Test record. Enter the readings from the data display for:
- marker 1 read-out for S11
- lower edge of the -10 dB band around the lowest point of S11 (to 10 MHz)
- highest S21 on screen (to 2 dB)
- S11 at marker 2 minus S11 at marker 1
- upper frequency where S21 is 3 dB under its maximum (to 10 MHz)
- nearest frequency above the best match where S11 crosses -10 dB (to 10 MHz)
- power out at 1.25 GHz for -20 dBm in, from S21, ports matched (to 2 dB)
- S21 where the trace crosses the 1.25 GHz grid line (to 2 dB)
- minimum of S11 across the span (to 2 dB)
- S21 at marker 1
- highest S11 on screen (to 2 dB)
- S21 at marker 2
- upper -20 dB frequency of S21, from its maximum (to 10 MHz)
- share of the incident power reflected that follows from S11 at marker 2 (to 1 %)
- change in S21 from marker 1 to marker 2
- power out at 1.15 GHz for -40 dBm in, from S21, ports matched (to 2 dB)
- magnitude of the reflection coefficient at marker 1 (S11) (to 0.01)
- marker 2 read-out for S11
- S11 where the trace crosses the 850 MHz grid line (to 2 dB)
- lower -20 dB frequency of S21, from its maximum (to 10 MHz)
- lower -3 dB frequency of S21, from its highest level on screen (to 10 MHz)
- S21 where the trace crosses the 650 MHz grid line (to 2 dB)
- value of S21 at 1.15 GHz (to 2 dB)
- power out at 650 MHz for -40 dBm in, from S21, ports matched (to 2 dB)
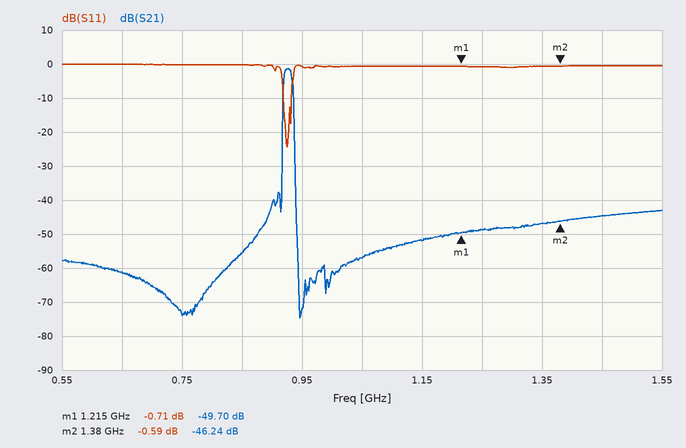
-0.71 dB
920 MHz
-2 dB
0.12 dB
930 MHz
930 MHz
-68 dBm
-48 dB
-24 dB
-49.70 dB
0 dB
-46.24 dB
940 MHz
87 %
3.46 dB
-92 dBm
0.92
-0.59 dB
0 dB
920 MHz
920 MHz
-62 dB
-52 dB
-102 dBm
